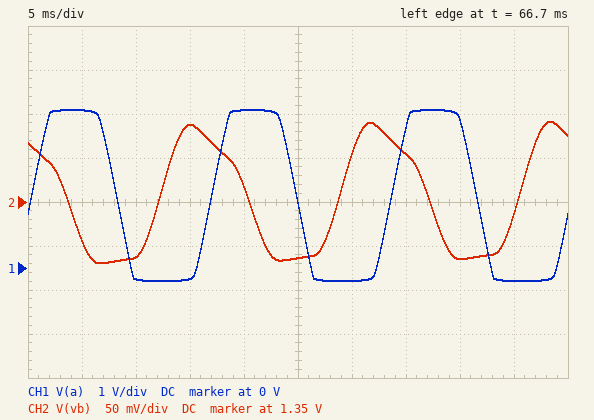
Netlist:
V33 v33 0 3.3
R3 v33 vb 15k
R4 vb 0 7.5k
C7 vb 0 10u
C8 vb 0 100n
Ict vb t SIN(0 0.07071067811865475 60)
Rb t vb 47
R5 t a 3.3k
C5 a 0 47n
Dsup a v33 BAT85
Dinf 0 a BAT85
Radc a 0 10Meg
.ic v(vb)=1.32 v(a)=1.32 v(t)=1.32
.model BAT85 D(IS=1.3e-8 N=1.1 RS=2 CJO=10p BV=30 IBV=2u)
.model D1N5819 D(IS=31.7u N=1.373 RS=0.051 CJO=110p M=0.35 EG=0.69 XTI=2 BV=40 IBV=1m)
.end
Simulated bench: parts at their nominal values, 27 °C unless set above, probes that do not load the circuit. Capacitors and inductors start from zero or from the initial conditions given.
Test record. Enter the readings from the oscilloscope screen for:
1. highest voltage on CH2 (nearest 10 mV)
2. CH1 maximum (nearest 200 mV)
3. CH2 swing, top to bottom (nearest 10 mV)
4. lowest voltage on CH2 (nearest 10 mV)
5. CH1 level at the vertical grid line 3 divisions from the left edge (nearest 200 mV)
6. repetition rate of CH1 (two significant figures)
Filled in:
1.44 V
3.6 V
160 mV
1.28 V
-200 mV
60 Hz
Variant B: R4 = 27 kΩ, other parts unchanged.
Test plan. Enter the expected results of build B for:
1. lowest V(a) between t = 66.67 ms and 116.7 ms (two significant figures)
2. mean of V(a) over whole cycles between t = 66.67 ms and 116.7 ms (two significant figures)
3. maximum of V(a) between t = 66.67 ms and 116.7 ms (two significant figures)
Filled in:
-290 mV
1.7 V
3.6 V
